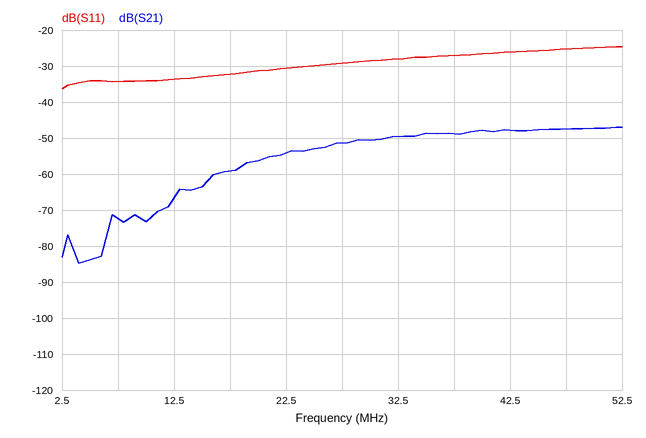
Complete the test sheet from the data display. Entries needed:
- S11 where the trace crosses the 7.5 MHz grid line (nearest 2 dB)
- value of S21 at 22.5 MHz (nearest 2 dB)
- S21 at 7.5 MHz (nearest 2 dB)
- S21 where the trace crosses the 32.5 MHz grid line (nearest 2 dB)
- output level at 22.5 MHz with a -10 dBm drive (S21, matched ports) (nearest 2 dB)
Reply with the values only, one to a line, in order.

-34 dB
-54 dB
-72 dB
-50 dB
-64 dBm
